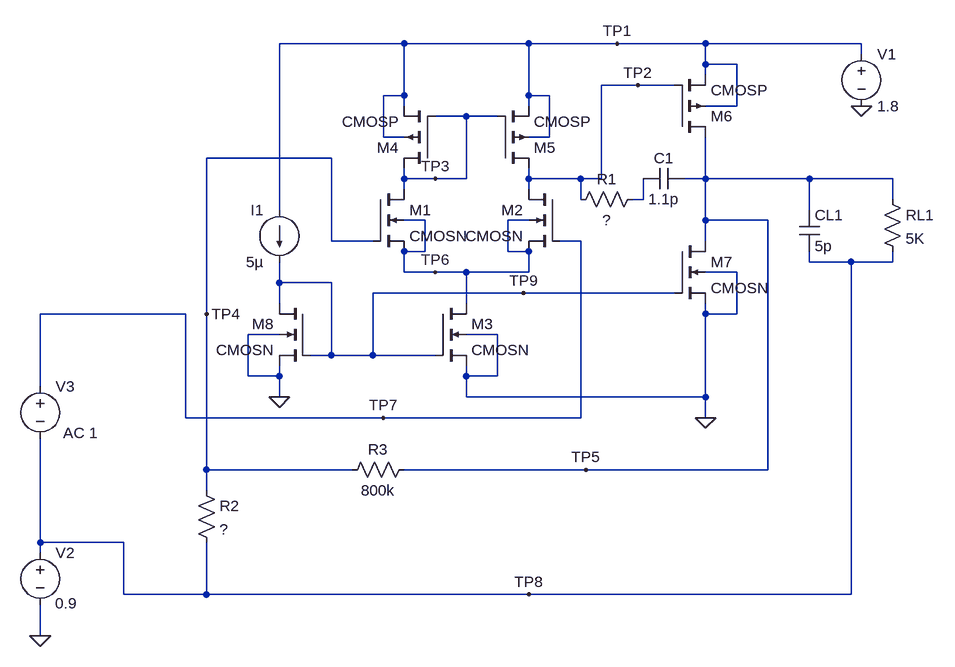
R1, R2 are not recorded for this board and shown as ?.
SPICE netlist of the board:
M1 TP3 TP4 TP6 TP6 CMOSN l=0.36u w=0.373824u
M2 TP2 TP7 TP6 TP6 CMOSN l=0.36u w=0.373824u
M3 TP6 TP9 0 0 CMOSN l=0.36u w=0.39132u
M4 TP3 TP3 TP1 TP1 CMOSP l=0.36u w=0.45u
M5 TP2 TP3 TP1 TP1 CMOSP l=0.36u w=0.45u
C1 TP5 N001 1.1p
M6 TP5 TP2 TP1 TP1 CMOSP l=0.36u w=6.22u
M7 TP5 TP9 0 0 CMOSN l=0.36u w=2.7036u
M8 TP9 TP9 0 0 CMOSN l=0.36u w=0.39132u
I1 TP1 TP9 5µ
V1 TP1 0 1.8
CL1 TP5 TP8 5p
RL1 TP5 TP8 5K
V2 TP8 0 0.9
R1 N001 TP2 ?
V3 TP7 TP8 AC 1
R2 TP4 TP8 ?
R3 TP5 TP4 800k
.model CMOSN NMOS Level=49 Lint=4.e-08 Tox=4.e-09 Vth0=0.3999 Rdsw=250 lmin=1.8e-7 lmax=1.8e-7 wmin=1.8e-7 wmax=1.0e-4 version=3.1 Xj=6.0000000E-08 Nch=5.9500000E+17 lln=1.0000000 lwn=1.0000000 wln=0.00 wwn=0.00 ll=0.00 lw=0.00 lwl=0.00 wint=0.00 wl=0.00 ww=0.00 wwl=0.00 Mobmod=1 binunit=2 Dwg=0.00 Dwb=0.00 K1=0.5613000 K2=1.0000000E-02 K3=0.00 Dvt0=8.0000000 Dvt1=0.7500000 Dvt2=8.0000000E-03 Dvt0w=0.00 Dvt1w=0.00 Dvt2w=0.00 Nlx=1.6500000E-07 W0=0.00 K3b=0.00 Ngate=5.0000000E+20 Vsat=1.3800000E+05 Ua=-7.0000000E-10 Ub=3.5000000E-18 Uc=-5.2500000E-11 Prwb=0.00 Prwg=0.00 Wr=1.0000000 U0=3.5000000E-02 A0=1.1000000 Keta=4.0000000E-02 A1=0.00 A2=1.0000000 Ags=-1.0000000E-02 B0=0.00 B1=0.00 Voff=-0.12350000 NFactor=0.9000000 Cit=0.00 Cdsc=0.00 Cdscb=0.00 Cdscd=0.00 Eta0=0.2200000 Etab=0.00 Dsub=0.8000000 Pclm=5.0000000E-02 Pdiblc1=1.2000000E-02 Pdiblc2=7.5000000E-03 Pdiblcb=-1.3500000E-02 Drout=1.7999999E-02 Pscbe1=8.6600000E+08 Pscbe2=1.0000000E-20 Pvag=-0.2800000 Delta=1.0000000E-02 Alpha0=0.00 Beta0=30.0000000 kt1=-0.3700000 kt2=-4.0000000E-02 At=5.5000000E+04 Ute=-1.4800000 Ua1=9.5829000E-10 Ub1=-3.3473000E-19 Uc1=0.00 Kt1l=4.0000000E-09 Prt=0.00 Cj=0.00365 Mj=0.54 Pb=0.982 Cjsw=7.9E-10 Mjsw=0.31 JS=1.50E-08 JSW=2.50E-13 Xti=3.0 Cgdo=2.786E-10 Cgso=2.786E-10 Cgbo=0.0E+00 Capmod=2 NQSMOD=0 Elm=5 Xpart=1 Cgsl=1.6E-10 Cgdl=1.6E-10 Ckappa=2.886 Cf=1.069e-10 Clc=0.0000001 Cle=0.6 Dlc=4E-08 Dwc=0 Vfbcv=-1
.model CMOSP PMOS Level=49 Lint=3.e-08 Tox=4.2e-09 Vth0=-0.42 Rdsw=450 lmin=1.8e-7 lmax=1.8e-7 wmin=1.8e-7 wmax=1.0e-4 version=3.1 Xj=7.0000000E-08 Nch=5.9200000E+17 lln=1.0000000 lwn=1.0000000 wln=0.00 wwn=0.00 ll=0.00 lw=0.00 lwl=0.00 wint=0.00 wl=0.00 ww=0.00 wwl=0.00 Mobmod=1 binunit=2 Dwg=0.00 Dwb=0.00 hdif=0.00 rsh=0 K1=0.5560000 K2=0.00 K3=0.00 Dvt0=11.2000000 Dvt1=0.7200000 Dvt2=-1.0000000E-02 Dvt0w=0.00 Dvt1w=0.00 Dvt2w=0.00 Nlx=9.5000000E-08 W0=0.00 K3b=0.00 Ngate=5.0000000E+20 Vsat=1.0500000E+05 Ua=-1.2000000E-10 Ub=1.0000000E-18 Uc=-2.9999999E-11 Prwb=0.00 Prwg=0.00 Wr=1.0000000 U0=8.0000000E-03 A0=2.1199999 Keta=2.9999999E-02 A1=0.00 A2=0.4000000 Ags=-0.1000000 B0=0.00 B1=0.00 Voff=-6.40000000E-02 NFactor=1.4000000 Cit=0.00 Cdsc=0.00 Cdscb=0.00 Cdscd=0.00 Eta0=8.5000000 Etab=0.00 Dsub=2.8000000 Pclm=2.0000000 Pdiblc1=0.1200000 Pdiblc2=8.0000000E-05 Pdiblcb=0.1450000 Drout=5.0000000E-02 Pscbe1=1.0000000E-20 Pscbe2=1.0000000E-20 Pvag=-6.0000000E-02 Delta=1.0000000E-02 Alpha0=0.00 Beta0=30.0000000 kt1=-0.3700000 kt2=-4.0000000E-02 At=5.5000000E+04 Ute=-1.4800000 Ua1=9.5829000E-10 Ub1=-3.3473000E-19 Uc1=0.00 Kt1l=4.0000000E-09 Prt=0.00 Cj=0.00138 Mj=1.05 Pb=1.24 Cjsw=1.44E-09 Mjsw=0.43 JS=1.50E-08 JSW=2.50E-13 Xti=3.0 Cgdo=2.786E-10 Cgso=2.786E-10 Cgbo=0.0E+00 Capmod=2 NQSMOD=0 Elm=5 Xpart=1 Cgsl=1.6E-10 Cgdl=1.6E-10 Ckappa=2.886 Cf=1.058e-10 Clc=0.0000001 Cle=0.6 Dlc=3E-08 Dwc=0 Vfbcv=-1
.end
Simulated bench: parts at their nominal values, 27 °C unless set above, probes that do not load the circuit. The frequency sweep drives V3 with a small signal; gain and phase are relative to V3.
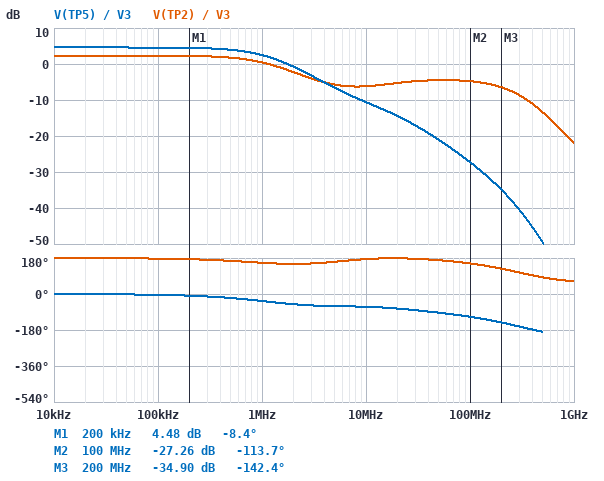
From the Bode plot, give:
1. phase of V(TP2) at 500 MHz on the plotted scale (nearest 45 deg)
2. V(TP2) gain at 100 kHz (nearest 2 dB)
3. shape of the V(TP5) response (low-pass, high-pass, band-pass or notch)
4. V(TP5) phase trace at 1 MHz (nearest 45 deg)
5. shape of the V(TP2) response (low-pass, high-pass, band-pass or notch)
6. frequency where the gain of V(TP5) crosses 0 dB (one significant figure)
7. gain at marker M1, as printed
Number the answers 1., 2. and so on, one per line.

1. 90 deg
2. 2 dB
3. low-pass
4. -45 deg
5. low-pass
6. 2 MHz
7. 4.48 dB
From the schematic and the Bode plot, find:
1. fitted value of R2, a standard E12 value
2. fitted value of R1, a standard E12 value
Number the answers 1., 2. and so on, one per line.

1. 1 MΩ
2. 22 kΩ
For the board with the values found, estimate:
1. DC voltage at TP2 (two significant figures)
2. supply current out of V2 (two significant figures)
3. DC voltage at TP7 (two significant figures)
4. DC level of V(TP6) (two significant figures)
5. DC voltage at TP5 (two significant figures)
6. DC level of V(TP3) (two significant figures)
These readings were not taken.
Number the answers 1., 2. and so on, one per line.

1. 1.1 V
2. 150 nA
3. 900 mV
4. 290 mV
5. 900 mV
6. 1.1 V
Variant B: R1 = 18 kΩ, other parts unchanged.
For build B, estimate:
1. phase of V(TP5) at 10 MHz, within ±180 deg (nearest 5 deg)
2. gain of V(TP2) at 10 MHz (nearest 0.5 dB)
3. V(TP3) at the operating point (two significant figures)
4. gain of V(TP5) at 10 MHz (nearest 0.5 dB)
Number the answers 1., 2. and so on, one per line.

1. -70 deg
2. -7.0 dB
3. 1.1 V
4. -11.5 dB
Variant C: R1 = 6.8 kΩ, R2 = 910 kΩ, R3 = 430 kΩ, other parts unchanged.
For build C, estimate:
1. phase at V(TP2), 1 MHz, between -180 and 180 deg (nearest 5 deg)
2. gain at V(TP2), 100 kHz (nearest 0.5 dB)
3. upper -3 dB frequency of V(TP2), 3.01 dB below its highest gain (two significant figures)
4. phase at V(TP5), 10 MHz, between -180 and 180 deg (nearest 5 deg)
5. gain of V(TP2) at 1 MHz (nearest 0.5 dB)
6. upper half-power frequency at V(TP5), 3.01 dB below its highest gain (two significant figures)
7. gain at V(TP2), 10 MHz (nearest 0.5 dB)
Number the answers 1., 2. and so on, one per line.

1. 160 deg
2. 0.5 dB
3. 2.0 MHz
4. -105 deg
5. -0.5 dB
6. 1.8 MHz
7. -9.0 dB
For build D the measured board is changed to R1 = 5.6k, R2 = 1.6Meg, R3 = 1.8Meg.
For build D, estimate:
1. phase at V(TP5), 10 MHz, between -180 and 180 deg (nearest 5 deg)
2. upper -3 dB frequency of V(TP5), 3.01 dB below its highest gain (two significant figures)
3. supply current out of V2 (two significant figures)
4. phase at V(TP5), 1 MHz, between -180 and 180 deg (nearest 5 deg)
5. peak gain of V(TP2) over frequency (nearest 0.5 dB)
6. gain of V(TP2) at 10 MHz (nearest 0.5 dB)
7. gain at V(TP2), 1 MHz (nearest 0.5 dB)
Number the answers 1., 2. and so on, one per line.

1. -110 deg
2. 1.2 MHz
3. 170 nA
4. -40 deg
5. 3.5 dB
6. -9.5 dB
7. 1.5 dB
